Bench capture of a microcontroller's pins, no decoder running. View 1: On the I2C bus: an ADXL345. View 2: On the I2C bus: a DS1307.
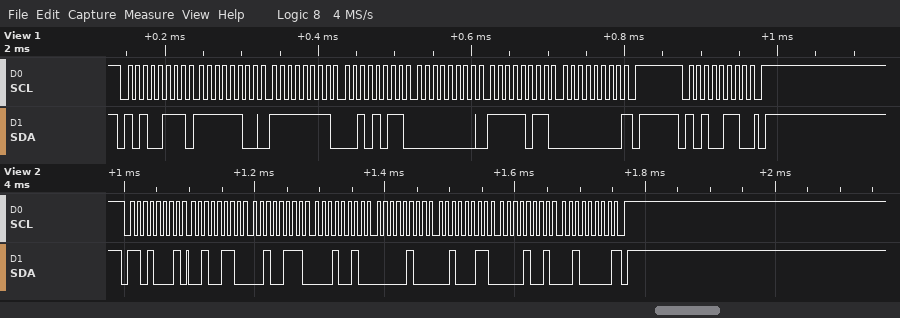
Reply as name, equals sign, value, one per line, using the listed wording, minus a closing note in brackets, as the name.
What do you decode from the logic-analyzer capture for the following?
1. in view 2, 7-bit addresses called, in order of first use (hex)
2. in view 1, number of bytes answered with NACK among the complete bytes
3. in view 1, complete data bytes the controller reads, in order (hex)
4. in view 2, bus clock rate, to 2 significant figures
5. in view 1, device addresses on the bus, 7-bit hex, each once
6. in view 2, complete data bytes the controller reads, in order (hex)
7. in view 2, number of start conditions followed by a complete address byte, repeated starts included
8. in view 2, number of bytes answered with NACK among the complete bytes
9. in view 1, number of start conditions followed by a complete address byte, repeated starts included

in view 2, 7-bit addresses called, in order of first use = 0x68
in view 1, number of bytes answered with NACK among the complete bytes = 1
in view 1, complete data bytes the controller reads, in order = FC FF 2B 00 FB 00
in view 2, bus clock rate, to 2 significant figures = 100 kHz
in view 1, device addresses on the bus, 7-bit hex, each once = 0x53
in view 2, complete data bytes the controller reads, in order = 26 27 12 04 23 09 20
in view 2, number of start conditions followed by a complete address byte, repeated starts included = 1
in view 2, number of bytes answered with NACK among the complete bytes = 1
in view 1, number of start conditions followed by a complete address byte, repeated starts included = 2
